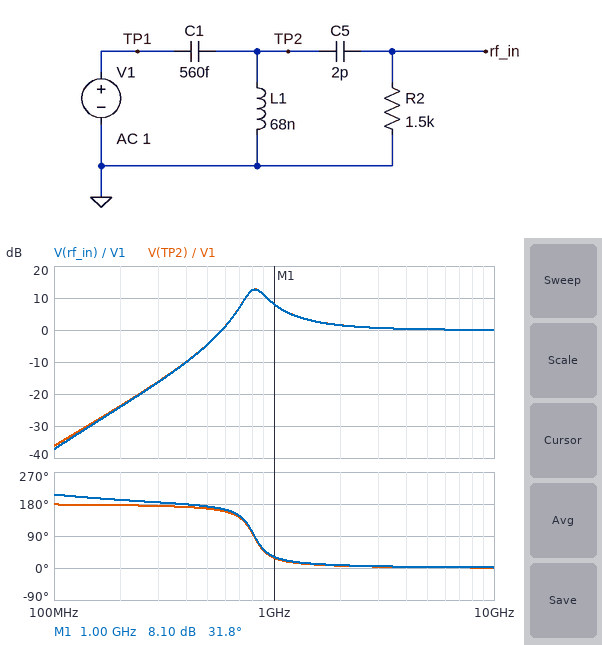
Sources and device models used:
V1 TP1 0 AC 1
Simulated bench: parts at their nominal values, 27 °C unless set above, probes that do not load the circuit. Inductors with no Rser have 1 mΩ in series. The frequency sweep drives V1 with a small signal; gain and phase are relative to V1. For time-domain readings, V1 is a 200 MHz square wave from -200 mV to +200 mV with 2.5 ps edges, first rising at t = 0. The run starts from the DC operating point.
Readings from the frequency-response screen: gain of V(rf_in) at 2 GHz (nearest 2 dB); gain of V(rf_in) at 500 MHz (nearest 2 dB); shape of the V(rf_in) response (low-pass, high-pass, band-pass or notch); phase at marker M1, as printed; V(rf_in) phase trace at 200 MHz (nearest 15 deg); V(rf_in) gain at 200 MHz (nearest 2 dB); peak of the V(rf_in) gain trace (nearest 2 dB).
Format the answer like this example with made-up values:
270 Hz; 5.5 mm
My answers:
2 dB; -4 dB; high-pass; 31.8 deg; 195 deg; -24 dB; 12 dB
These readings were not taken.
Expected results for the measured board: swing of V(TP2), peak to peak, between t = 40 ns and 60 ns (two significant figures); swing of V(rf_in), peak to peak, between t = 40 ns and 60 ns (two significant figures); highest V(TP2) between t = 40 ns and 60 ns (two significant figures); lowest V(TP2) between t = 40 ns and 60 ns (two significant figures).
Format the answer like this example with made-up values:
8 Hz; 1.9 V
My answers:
650 mV; 650 mV; 330 mV; -330 mV
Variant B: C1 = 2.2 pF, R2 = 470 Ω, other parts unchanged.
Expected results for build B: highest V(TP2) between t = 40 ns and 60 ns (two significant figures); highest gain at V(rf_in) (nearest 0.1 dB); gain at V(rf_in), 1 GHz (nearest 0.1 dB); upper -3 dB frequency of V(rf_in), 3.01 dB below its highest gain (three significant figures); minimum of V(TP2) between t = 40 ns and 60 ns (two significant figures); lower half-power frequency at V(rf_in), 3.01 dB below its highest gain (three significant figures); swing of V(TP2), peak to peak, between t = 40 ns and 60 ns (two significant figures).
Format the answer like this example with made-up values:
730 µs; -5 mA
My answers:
290 mV; 8.8 dB; 1.1 dB; 492 MHz; -290 mV; 340 MHz; 580 mV
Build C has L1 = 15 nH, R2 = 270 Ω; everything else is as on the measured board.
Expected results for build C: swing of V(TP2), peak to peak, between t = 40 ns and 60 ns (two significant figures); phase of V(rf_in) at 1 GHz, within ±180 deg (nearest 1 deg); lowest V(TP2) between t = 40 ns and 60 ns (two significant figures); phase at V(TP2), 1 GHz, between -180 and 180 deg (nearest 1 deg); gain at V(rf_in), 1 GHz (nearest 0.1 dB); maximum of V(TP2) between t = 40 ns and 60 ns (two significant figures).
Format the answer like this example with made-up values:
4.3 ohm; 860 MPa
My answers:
790 mV; 167 deg; -400 mV; 151 deg; -6.3 dB; 400 mV
